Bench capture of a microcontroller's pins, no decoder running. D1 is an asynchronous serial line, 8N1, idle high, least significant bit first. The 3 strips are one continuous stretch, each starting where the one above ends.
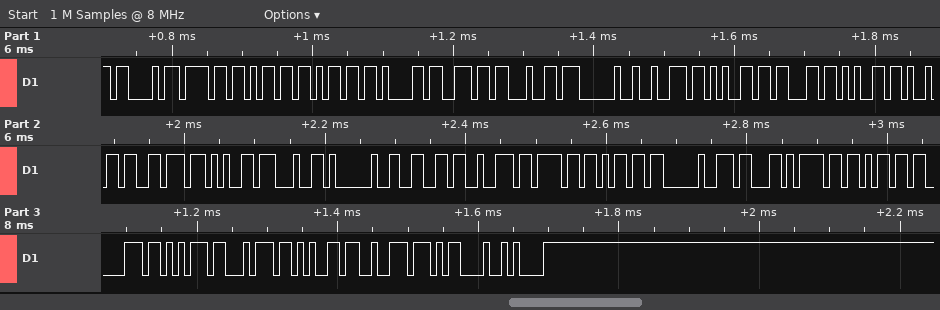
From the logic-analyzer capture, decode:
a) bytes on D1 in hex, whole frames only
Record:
43 6F 6D 6D 61 6E 64 20 72 65 63 65 69 76 65 64 20 66 72 6F 6D 20 63 6F 6D 70 75 74 65 72 0D 0A
